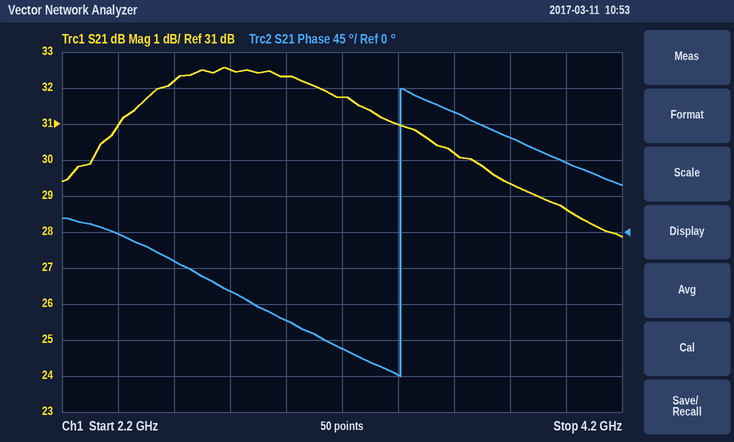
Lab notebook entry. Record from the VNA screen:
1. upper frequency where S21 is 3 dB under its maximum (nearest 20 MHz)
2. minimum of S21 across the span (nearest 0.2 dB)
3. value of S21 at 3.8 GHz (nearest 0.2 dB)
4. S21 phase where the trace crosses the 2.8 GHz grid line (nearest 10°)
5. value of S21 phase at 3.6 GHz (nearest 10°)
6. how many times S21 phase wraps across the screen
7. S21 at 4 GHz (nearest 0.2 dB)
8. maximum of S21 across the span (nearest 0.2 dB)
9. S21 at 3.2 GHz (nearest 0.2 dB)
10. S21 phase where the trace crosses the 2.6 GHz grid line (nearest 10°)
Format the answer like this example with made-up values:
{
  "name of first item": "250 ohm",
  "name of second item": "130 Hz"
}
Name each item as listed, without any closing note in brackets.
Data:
{
  "upper frequency where S21 is 3 dB under its maximum": "3.74 GHz",
  "minimum of S21 across the span": "27.8 dB",
  "value of S21 at 3.8 GHz": "29.4 dB",
  "S21 phase where the trace crosses the 2.8 GHz grid line": "-70°",
  "value of S21 phase at 3.6 GHz": "150°",
  "how many times S21 phase wraps across the screen": "1",
  "S21 at 4 GHz": "28.6 dB",
  "maximum of S21 across the span": "32.6 dB",
  "S21 at 3.2 GHz": "31.8 dB",
  "S21 phase where the trace crosses the 2.6 GHz grid line": "-40°"
}
